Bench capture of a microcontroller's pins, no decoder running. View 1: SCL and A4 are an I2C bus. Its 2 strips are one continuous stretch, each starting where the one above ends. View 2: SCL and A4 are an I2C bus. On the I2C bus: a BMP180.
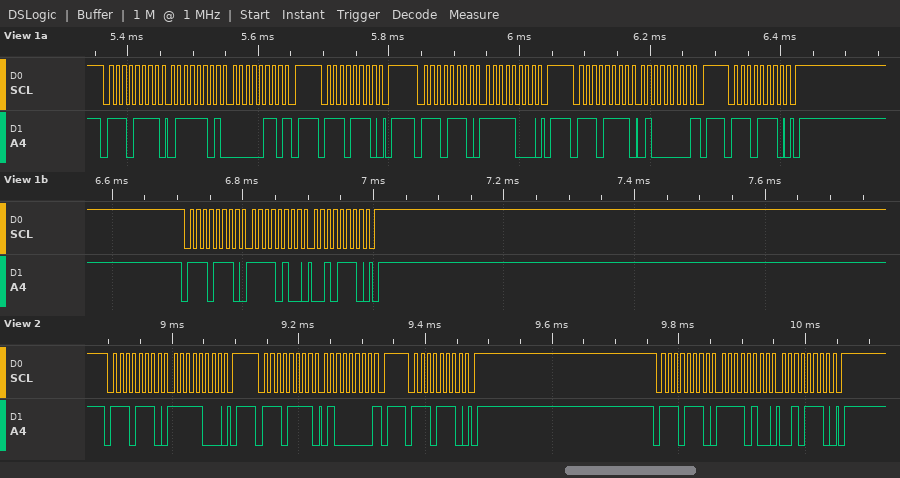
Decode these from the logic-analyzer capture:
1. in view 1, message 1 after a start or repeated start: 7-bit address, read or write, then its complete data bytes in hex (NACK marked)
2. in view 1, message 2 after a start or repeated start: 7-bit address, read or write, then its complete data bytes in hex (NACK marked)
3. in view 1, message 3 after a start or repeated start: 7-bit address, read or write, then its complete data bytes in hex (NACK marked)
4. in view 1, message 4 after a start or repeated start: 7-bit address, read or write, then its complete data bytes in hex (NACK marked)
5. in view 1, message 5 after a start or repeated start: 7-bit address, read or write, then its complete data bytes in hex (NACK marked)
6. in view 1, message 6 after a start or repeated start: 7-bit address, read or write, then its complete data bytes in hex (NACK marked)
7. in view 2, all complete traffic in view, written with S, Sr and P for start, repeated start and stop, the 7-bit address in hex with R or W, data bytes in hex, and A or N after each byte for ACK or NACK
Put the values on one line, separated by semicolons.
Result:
0x77 read: 7D 06 NACK; 0x77 write; 0x77 write: F8; 0x77 read: 40 NACK; 0x77 write; 0x77 write: F4 2E; S 77W A F8 A P S 77R A 40 N P S 77W A P S 77W A F4 A 2E A P
